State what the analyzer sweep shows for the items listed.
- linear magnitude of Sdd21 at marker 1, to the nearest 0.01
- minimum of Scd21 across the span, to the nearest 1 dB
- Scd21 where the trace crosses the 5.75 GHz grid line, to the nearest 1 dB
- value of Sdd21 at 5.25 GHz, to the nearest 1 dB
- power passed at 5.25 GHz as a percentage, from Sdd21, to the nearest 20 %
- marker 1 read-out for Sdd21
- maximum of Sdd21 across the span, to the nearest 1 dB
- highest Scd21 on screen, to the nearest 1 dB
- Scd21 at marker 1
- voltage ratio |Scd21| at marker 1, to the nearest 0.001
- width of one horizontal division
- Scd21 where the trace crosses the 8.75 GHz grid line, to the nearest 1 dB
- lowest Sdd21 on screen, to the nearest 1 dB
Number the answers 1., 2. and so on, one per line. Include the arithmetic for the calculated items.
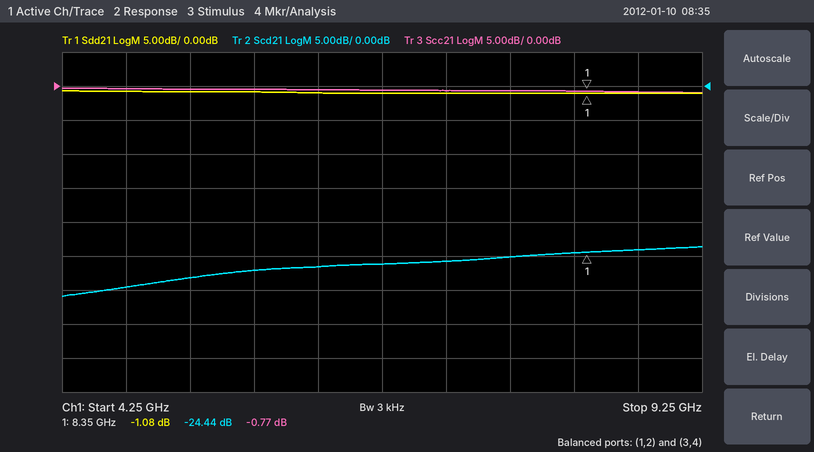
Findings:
1. 10^(-1.08/20) ≈ 0.88
2. -31 dB
3. -27 dB
4. -1 dB
5. 10^(-1/10) ≈ 79.4 %, so 80 % to the nearest 20 %
6. -1.08 dB
7. -1 dB
8. -24 dB
9. -24.44 dB
10. 10^(-24.44/20) ≈ 0.060
11. 500 MHz
12. -24 dB
13. -1 dB
